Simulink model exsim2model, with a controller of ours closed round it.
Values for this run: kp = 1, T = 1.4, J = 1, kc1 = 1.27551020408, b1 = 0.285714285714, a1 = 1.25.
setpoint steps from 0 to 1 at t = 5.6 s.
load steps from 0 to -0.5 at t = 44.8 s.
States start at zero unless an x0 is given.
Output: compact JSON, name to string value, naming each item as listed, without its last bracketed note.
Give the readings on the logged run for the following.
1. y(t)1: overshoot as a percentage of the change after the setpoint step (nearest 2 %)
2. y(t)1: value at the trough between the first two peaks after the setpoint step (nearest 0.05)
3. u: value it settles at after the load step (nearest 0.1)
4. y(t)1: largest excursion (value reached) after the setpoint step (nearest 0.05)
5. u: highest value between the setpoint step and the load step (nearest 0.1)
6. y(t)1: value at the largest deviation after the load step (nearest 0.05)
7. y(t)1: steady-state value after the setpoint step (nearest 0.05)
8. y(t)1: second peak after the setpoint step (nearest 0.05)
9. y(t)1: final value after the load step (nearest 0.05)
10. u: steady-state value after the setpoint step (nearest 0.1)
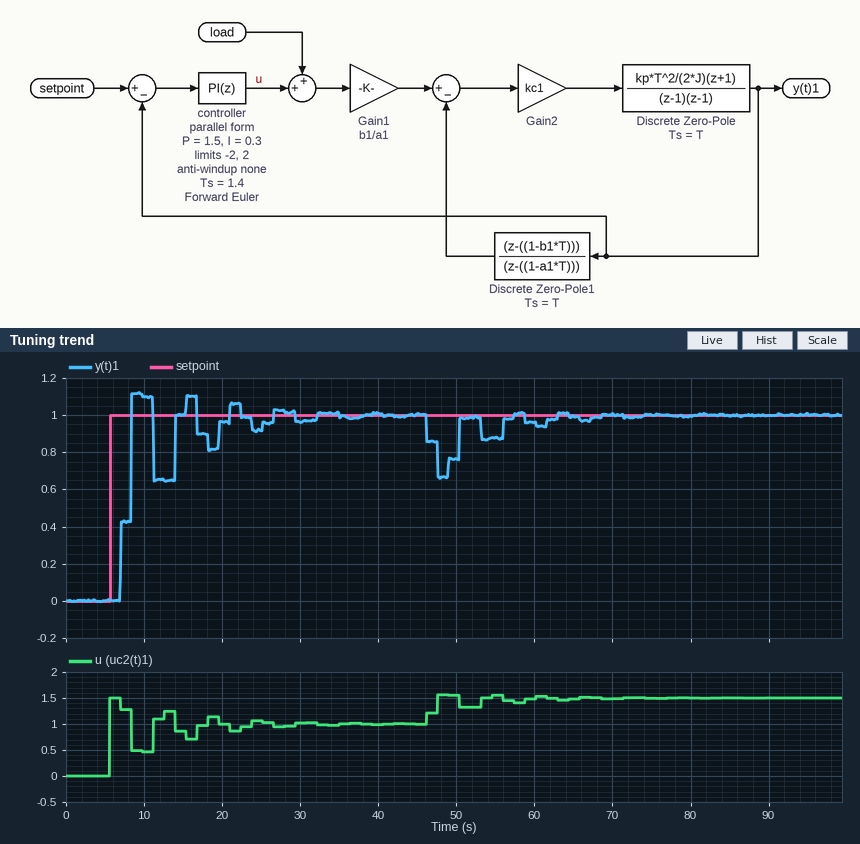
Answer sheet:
{"y(t)1: overshoot as a percentage of the change after the setpoint step": "12 %", "y(t)1: value at the trough between the first two peaks after the setpoint step": "0.65", "u: value it settles at after the load step": "1.5", "y(t)1: largest excursion (value reached) after the setpoint step": "1.10", "u: highest value between the setpoint step and the load step": "1.5", "y(t)1: value at the largest deviation after the load step": "0.65", "y(t)1: steady-state value after the setpoint step": "1.00", "y(t)1: second peak after the setpoint step": "1.10", "y(t)1: final value after the load step": "1.00", "u: steady-state value after the setpoint step": "1.0"}
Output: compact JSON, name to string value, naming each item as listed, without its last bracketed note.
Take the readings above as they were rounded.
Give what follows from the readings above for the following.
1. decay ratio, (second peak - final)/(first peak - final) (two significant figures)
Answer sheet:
{"decay ratio, (second peak - final)/(first peak - final)": "1.0"}
